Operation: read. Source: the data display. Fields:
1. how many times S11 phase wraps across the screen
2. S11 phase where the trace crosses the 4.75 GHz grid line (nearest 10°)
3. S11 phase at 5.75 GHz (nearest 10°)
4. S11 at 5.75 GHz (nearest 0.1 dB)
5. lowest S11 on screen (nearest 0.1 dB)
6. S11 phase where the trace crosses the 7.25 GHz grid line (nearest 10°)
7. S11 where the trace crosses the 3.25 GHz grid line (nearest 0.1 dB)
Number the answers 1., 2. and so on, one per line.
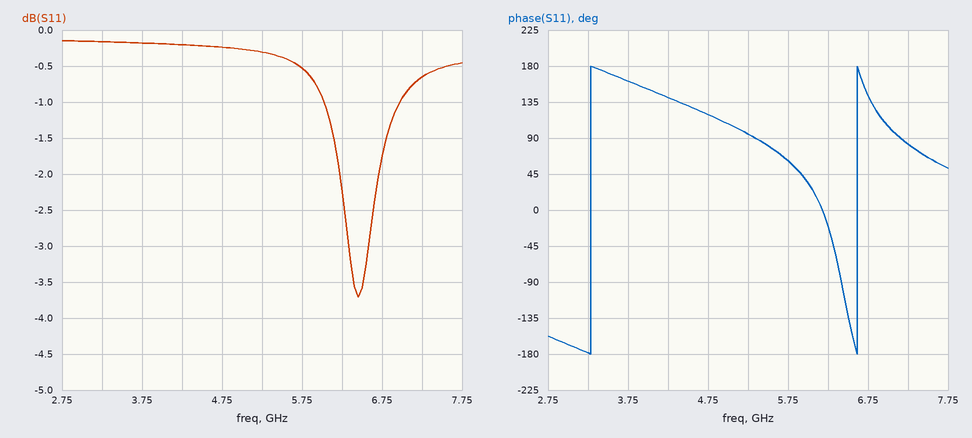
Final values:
1. 2
2. 120°
3. 60°
4. -0.5 dB
5. -3.7 dB
6. 80°
7. -0.2 dB
